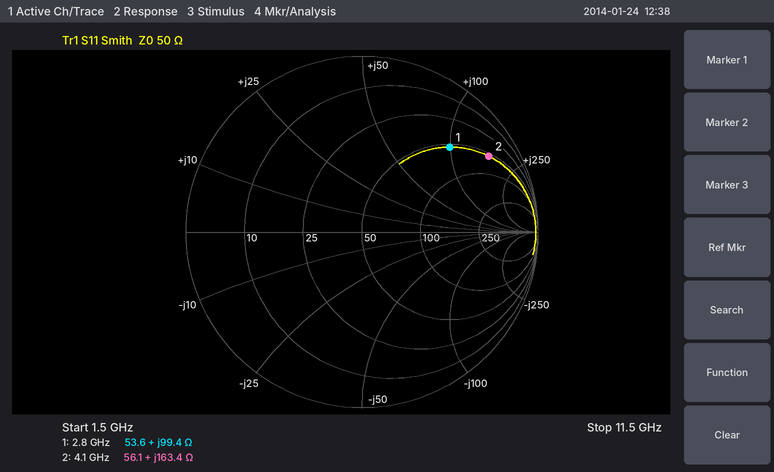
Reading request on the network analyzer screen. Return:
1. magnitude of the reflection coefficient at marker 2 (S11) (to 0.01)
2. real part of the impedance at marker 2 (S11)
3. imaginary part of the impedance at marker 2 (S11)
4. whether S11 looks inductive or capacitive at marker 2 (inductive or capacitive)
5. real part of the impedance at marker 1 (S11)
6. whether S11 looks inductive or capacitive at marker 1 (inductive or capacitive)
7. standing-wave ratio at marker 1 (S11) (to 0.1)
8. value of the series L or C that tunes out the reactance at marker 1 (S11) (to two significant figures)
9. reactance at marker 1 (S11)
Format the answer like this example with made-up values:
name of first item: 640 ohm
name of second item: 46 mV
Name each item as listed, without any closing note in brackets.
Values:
magnitude of the reflection coefficient at marker 2 (S11): 0.84
real part of the impedance at marker 2: 56.1 Ω
imaginary part of the impedance at marker 2: +163.4 Ω
whether S11 looks inductive or capacitive at marker 2: inductive
real part of the impedance at marker 1: 53.6 Ω
whether S11 looks inductive or capacitive at marker 1: inductive
standing-wave ratio at marker 1 (S11): 5.5
value of the series L or C that tunes out the reactance at marker 1 (S11): 570 fF
reactance at marker 1: +99.4 Ω
